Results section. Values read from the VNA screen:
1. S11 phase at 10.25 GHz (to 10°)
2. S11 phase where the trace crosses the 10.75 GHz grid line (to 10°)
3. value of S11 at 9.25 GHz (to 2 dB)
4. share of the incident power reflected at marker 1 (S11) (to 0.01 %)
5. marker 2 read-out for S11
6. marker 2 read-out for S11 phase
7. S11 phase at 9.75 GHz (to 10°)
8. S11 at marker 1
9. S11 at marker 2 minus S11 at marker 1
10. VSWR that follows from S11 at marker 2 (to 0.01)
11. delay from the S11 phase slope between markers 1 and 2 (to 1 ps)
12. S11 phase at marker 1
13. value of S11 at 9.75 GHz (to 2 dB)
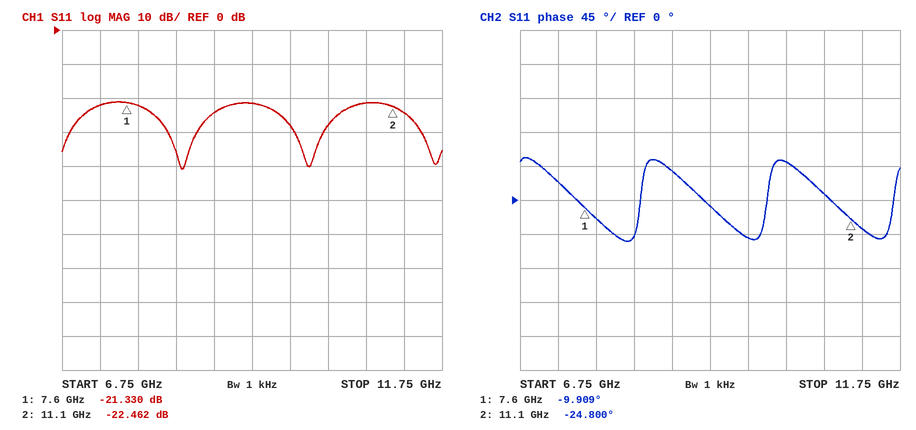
50°
10°
-22 dB
0.74 %
-22.462 dB
-24.800°
-50°
-21.330 dB
-1.132 dB
1.16
12 ps
-9.909°
-28 dB
